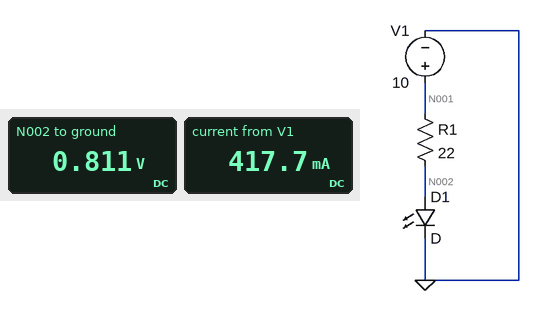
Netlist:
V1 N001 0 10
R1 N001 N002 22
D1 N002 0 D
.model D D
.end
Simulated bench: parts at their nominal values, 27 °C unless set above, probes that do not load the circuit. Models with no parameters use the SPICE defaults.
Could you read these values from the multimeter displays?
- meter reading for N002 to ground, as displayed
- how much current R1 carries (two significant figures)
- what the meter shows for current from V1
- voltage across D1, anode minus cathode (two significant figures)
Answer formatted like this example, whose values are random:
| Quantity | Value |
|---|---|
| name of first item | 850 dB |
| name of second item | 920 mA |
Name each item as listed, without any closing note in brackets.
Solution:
| Quantity | Value |
|---|---|
| meter reading for N002 to ground, as displayed | 0.811 V |
| how much current R1 carries | 420 mA |
| what the meter shows for current from V1 | 417.7 mA |
| voltage across D1, anode minus cathode | 810 mV |
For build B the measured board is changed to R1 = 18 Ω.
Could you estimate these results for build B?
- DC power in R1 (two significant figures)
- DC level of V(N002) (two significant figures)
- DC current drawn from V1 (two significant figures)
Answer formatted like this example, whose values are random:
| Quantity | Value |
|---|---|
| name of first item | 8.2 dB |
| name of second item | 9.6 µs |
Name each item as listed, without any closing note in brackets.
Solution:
| Quantity | Value |
|---|---|
| DC power in R1 | 4.7 W |
| DC level of V(N002) | 820 mV |
| DC current drawn from V1 | 510 mA |
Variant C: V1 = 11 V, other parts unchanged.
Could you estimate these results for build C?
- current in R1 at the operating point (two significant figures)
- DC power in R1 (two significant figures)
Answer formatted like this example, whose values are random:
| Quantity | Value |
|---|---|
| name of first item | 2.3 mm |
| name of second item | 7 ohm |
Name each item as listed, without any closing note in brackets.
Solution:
| Quantity | Value |
|---|---|
| current in R1 at the operating point | 460 mA |
| DC power in R1 | 4.7 W |
